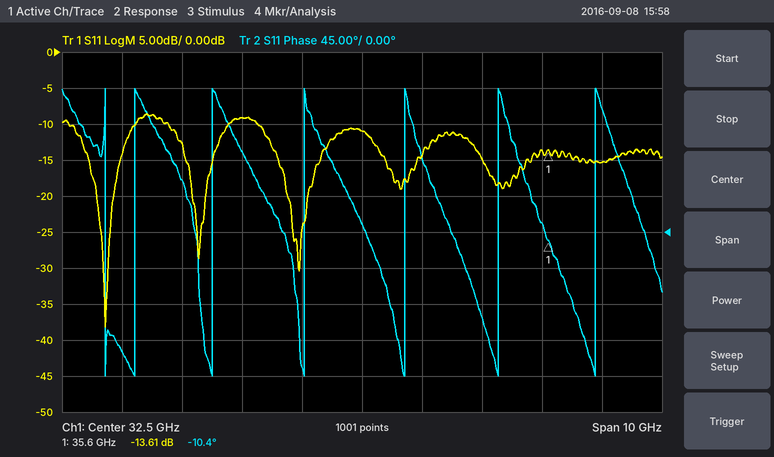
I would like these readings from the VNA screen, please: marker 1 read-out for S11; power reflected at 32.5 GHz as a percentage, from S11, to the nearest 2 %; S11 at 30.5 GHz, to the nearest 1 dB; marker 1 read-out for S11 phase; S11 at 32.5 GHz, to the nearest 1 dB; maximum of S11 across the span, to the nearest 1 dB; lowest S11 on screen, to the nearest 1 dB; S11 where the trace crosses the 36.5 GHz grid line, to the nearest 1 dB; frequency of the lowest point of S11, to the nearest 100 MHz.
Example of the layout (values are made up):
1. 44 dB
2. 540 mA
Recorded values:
1. -13.61 dB
2. 8 %
3. -9 dB
4. -10.4°
5. -11 dB
6. -9 dB
7. -38 dB
8. -15 dB
9. 28.2 GHz
